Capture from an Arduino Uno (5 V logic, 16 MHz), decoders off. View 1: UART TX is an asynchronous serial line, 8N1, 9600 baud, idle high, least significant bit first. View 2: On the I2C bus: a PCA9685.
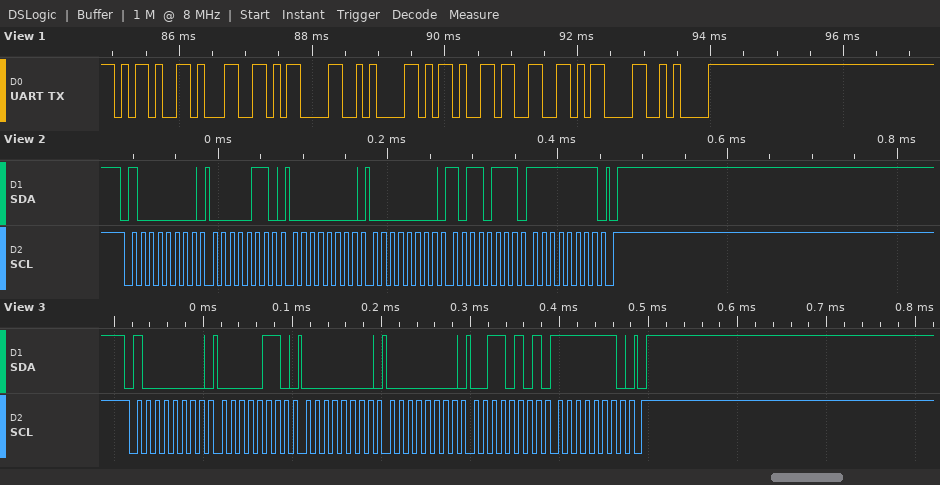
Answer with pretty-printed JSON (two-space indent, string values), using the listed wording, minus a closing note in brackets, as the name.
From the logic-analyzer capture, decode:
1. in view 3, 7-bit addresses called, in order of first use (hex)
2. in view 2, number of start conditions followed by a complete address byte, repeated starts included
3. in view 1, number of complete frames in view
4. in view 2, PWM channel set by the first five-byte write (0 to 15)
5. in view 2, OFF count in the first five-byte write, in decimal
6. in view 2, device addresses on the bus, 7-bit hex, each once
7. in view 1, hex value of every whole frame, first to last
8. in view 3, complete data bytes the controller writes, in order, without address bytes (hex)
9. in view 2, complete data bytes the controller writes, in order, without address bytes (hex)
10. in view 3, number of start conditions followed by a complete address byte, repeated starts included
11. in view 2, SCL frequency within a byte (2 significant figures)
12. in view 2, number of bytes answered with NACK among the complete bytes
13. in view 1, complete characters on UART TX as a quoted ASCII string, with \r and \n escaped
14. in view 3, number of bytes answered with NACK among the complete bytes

{
  "in view 3, 7-bit addresses called, in order of first use": "0x40",
  "in view 2, number of start conditions followed by a complete address byte, repeated starts included": "1",
  "in view 1, number of complete frames in view": "8",
  "in view 2, PWM channel set by the first five-byte write": "0",
  "in view 2, OFF count in the first five-byte write, in decimal": "65463",
  "in view 2, device addresses on the bus, 7-bit hex, each once": "0x40",
  "in view 1, hex value of every whole frame, first to last": "2D 31 0D 0A 2D 33 0D 0A",
  "in view 3, complete data bytes the controller writes, in order, without address bytes": "06 00 00 35 FE",
  "in view 2, complete data bytes the controller writes, in order, without address bytes": "06 00 00 B7 FF",
  "in view 3, number of start conditions followed by a complete address byte, repeated starts included": "1",
  "in view 2, SCL frequency within a byte": "100 kHz",
  "in view 2, number of bytes answered with NACK among the complete bytes": "0",
  "in view 1, complete characters on UART TX as a quoted ASCII string, with \\r and \\n escaped": "\"-1\\r\\n-3\\r\\n\"",
  "in view 3, number of bytes answered with NACK among the complete bytes": "0"
}
